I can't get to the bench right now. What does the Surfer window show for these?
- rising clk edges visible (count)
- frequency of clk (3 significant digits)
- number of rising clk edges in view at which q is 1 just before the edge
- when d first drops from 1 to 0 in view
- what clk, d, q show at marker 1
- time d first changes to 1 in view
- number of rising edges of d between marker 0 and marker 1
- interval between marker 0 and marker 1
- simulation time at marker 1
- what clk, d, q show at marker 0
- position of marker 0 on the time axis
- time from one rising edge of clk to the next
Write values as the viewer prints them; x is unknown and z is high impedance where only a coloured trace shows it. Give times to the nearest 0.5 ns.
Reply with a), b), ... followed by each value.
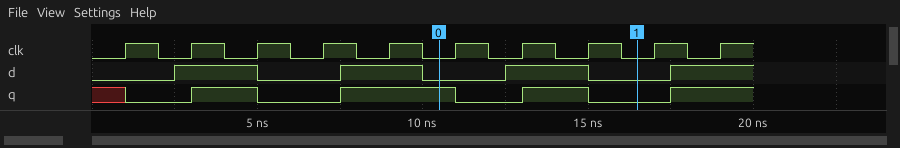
a) 10
b) 500 MHz
c) 5
d) 5 ns
e) clk=0, d=0, q=0
f) 2.5 ns
g) 1
h) 6 ns
i) 16.5 ns
j) clk=0, d=0, q=1
k) 10.5 ns
l) 2 ns
